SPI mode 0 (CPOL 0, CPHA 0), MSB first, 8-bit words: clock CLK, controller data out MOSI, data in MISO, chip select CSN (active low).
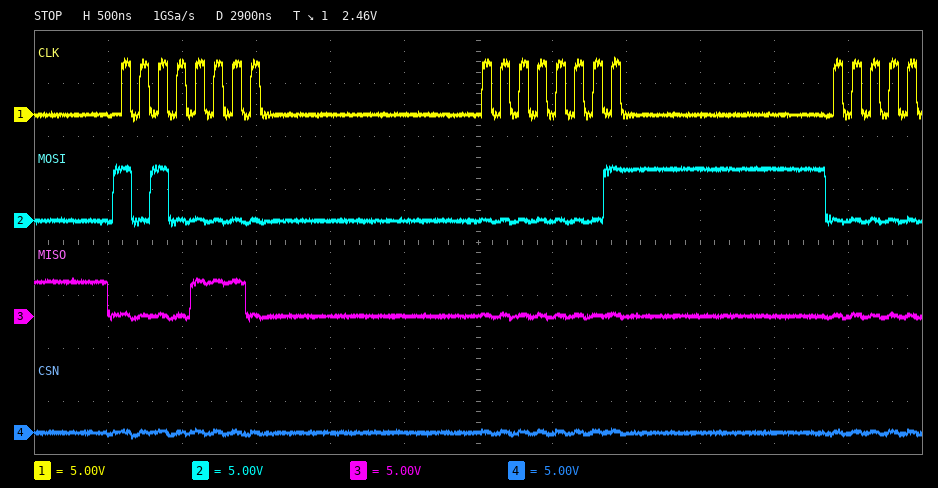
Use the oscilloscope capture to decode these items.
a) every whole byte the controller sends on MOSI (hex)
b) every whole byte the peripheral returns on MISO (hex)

A0 01
0E 00
